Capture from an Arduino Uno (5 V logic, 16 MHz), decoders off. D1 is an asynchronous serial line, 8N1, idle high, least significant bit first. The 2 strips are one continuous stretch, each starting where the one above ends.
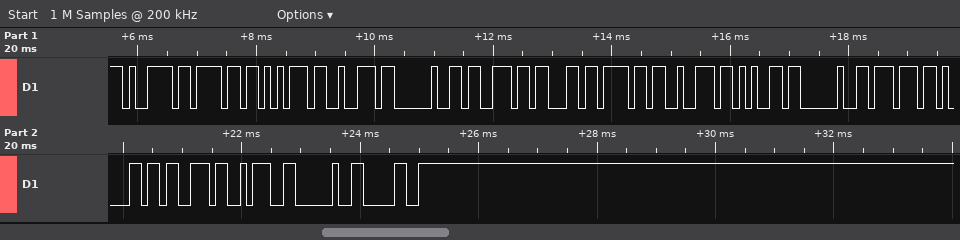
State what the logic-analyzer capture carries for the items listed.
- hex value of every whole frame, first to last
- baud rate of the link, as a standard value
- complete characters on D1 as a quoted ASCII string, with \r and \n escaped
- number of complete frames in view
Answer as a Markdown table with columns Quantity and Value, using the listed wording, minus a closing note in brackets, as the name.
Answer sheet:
| Quantity | Value |
|---|---|
| hex value of every whole frame, first to last | 79 6F 75 72 20 73 63 6F 72 65 20 77 61 73 3A 20 30 |
| baud rate of the link, as a standard value | 9600 baud |
| complete characters on D1 as a quoted ASCII string, with \r and \n escaped | "your score was: 0" |
| number of complete frames in view | 17 |
